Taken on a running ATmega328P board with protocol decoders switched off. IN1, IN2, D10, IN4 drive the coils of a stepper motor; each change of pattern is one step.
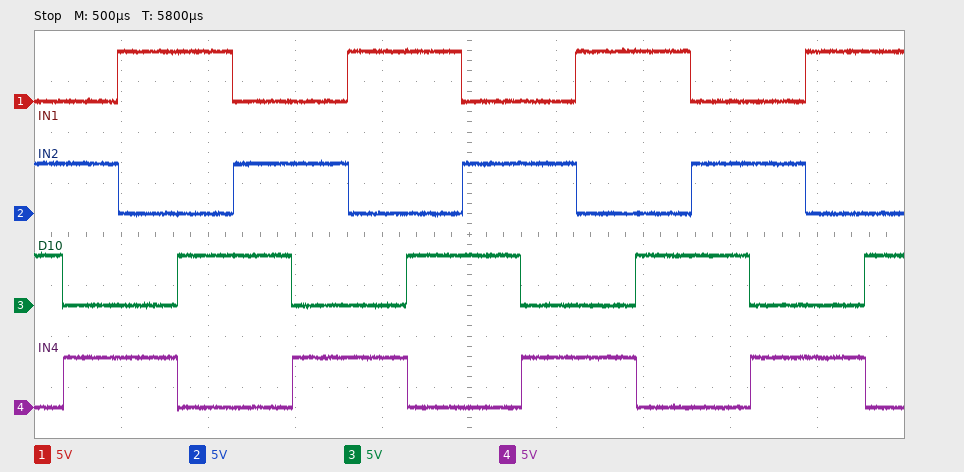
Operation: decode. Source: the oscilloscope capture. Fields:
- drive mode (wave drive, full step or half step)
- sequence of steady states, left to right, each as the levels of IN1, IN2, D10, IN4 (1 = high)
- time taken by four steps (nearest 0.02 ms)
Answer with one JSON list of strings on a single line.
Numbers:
["full step", "0110 0101 1001 1010 0110 0101 1001 1010 0110 0101 1001 1010 0110 0101 1001 1010", "1.32 ms"]
